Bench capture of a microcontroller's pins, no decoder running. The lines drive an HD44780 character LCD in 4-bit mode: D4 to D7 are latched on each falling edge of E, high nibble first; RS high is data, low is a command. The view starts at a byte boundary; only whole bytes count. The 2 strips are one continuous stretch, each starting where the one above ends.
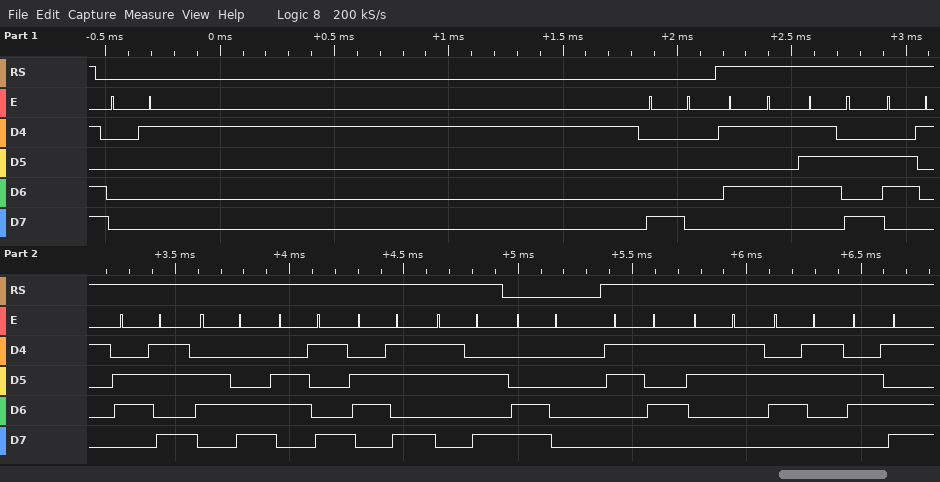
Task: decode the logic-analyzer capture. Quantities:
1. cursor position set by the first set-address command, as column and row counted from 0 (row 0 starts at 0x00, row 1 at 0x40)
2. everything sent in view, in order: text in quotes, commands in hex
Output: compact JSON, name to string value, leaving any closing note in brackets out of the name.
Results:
{"cursor position set by the first set-address command, as column and row counted from 0": "column 0, row 0", "everything sent in view, in order: text in quotes, commands in hex": "0x01 0x80 \"Uzaklik:\" 0xC0 \"53cm\""}
